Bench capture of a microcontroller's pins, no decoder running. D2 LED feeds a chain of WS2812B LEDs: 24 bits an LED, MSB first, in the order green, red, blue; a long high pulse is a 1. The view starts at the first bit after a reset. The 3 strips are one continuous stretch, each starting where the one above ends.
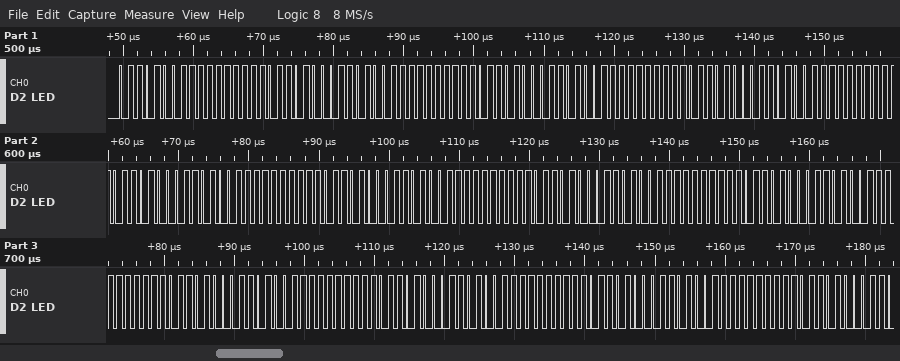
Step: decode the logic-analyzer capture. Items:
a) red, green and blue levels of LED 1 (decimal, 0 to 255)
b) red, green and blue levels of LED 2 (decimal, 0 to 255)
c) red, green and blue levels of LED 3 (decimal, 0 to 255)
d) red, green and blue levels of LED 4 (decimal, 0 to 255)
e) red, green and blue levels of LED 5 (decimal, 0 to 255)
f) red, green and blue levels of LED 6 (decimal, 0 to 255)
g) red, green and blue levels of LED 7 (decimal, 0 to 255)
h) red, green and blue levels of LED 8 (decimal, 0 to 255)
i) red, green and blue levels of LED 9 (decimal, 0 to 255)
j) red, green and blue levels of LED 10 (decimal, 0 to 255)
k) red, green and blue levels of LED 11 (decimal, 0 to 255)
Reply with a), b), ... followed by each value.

a) 255, 105, 180
b) 255, 105, 180
c) 255, 105, 180
d) 255, 105, 180
e) 255, 105, 180
f) 255, 105, 180
g) 255, 105, 180
h) 255, 105, 180
i) 255, 105, 180
j) 255, 105, 180
k) 255, 105, 180
